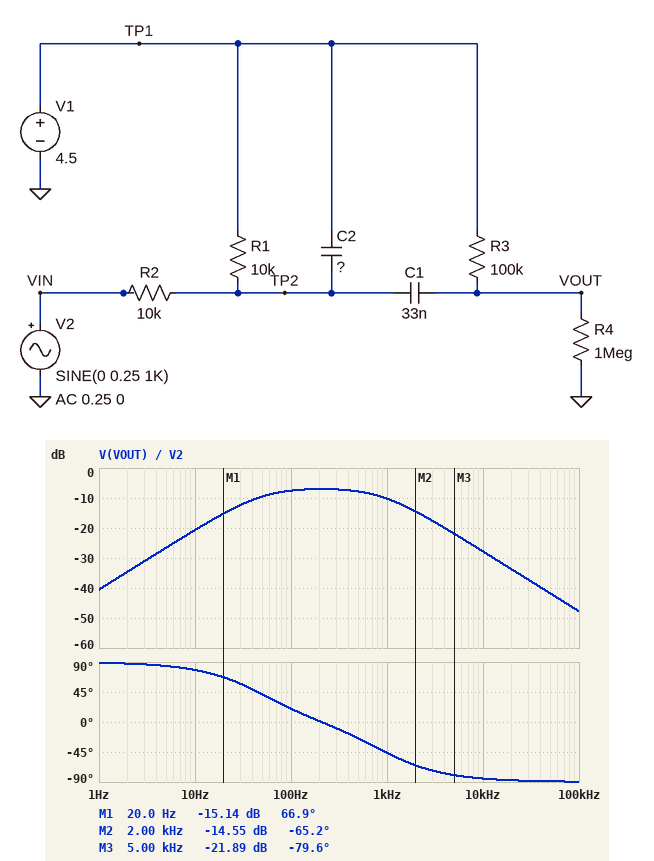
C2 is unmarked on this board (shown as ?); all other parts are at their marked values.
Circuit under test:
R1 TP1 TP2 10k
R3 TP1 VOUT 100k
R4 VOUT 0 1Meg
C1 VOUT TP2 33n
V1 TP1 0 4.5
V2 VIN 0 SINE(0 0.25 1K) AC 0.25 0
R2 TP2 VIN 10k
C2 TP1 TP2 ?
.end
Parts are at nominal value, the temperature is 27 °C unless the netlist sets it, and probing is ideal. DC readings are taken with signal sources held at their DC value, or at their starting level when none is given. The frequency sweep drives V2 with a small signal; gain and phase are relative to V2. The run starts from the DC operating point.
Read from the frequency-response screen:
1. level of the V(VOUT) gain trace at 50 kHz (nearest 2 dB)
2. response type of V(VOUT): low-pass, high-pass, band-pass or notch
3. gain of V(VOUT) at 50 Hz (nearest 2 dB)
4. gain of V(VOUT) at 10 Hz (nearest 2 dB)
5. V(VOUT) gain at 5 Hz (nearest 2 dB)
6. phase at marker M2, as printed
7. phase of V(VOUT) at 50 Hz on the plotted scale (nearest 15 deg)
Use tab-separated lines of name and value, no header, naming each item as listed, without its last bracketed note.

level of the V(VOUT) gain trace at 50 kHz	-42 dB
response type of V(VOUT): low-pass, high-pass, band-pass or notch	band-pass
gain of V(VOUT) at 50 Hz	-10 dB
gain of V(VOUT) at 10 Hz	-20 dB
V(VOUT) gain at 5 Hz	-26 dB
phase at marker M2, as printed	-65.2 deg
phase of V(VOUT) at 50 Hz on the plotted scale	45 deg
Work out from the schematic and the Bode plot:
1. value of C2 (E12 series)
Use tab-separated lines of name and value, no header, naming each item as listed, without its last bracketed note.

value of C2	39 nF
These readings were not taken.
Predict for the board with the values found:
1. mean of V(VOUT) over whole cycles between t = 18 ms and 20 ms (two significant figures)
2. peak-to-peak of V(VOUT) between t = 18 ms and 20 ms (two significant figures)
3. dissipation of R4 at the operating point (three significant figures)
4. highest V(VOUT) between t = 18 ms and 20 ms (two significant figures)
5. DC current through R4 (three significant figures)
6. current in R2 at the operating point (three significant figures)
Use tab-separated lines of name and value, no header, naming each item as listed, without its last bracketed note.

mean of V(VOUT) over whole cycles between t = 18 ms and 20 ms	4.1 V
peak-to-peak of V(VOUT) between t = 18 ms and 20 ms	150 mV
dissipation of R4 at the operating point	16.7 µW
highest V(VOUT) between t = 18 ms and 20 ms	4.2 V
DC current through R4	4.09 µA
current in R2 at the operating point	225 µA
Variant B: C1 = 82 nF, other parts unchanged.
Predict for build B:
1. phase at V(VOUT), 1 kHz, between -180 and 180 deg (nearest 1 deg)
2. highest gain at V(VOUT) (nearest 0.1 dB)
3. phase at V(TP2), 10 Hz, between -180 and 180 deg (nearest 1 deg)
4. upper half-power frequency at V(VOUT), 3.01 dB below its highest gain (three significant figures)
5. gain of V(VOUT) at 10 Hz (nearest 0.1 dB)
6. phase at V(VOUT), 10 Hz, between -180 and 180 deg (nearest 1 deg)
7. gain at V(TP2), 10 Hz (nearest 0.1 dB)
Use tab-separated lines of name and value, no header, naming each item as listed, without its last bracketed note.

phase at V(VOUT), 1 kHz, between -180 and 180 deg	-48 deg
highest gain at V(VOUT)	-6.7 dB
phase at V(TP2), 10 Hz, between -180 and 180 deg	-2 deg
upper half-power frequency at V(VOUT), 3.01 dB below its highest gain	902 Hz
gain of V(VOUT) at 10 Hz	-13.6 dB
phase at V(VOUT), 10 Hz, between -180 and 180 deg	63 deg
gain at V(TP2), 10 Hz	-6.1 dB
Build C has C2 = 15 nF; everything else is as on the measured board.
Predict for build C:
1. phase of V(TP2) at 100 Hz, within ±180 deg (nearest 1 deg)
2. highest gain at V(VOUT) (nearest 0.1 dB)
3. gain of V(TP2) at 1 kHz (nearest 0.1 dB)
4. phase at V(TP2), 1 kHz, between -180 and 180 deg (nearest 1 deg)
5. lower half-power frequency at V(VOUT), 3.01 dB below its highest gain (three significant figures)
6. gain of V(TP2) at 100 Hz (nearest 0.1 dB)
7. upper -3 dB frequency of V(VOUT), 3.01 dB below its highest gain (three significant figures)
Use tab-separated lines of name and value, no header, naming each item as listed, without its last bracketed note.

phase of V(TP2) at 100 Hz, within ±180 deg	-4 deg
highest gain at V(VOUT)	-6.7 dB
gain of V(TP2) at 1 kHz	-7.3 dB
phase at V(TP2), 1 kHz, between -180 and 180 deg	-24 deg
lower half-power frequency at V(VOUT), 3.01 dB below its highest gain	48.1 Hz
gain of V(TP2) at 100 Hz	-6.4 dB
upper -3 dB frequency of V(VOUT), 3.01 dB below its highest gain	2.34 kHz
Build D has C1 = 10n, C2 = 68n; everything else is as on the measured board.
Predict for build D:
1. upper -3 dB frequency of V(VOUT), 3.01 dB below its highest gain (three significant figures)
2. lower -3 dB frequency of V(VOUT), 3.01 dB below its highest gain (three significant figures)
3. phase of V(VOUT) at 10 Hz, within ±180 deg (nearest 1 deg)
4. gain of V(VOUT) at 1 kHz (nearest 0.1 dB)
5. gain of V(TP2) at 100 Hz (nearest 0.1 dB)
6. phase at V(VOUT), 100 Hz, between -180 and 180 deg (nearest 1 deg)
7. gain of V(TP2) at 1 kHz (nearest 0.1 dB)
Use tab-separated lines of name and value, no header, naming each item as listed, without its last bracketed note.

upper -3 dB frequency of V(VOUT), 3.01 dB below its highest gain	775 Hz
lower -3 dB frequency of V(VOUT), 3.01 dB below its highest gain	106 Hz
phase of V(VOUT) at 10 Hz, within ±180 deg	85 deg
gain of V(VOUT) at 1 kHz	-13.7 dB
gain of V(TP2) at 100 Hz	-6.4 dB
phase at V(VOUT), 100 Hz, between -180 and 180 deg	47 deg
gain of V(TP2) at 1 kHz	-13.6 dB
